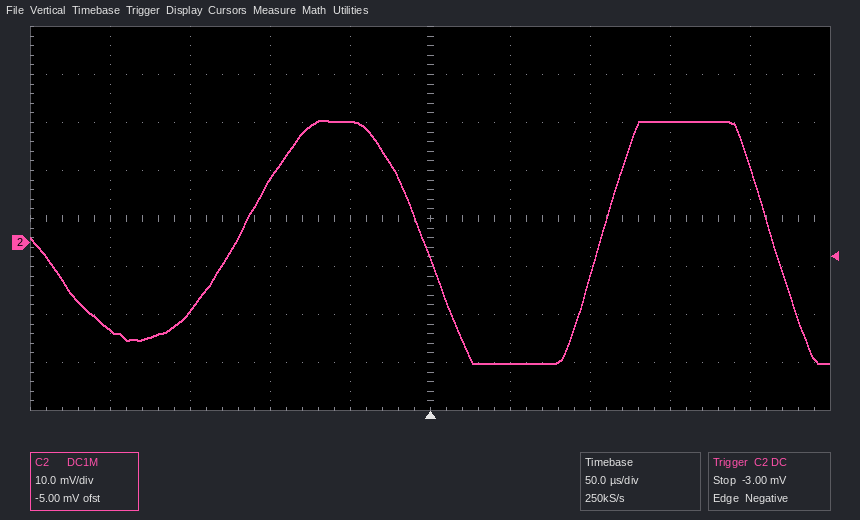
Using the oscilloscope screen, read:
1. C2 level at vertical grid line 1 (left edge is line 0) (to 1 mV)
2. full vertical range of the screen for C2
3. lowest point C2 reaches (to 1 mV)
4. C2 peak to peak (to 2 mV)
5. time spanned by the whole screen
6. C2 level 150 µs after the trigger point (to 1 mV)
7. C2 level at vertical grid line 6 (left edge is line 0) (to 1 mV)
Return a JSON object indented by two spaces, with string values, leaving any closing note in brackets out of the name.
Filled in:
{
  "C2 level at vertical grid line 1 (left edge is line 0)": "-18 mV",
  "full vertical range of the screen for C2": "80 mV",
  "lowest point C2 reaches": "-25 mV",
  "C2 peak to peak": "50 mV",
  "time spanned by the whole screen": "500 µs",
  "C2 level 150 µs after the trigger point": "25 mV",
  "C2 level at vertical grid line 6 (left edge is line 0)": "-25 mV"
}
